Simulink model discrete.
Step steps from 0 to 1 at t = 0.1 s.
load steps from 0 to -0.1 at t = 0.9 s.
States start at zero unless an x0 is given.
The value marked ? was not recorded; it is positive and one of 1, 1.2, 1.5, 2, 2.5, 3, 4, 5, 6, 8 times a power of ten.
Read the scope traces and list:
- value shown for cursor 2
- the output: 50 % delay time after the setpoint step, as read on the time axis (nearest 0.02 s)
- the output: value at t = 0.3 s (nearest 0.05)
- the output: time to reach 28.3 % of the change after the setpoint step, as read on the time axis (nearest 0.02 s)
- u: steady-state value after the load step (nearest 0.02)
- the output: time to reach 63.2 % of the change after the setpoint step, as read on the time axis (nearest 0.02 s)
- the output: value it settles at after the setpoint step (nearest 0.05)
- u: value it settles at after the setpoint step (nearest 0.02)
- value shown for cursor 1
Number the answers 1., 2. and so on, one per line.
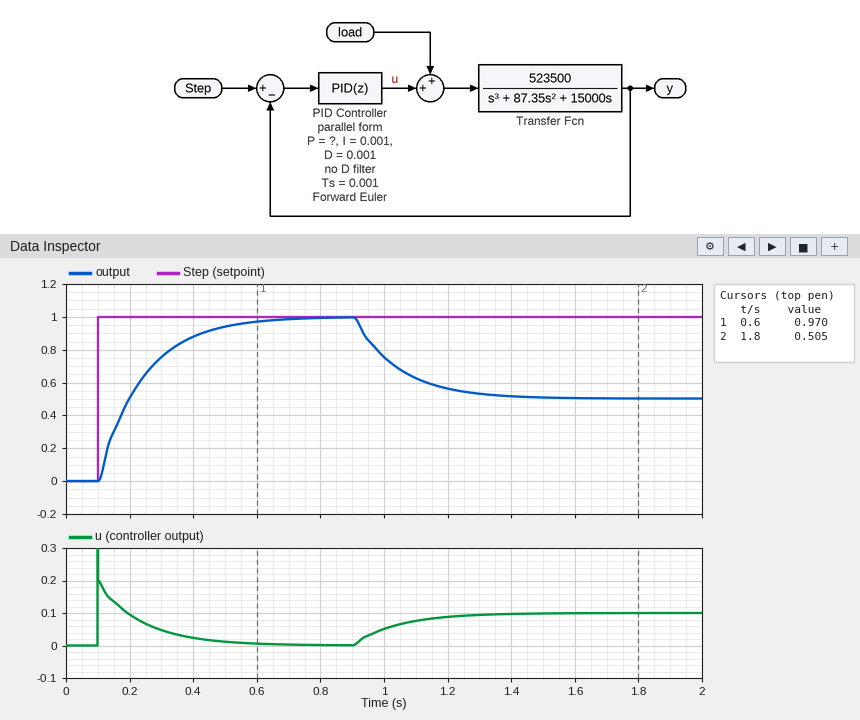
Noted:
1. 0.505
2. 0.20 s
3. 0.75
4. 0.14 s
5. 0.10
6. 0.24 s
7. 1.00
8. 0.00
9. 0.970
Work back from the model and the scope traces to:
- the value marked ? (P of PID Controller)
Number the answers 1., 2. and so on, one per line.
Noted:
1. 0.2
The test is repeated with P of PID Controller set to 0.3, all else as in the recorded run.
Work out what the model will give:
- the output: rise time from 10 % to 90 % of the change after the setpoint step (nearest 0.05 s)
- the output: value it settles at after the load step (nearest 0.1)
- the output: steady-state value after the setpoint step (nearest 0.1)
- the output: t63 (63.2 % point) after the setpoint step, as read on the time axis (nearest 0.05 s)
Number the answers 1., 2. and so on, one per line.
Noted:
1. 0.20 s
2. 0.7
3. 1.0
4. 0.20 s
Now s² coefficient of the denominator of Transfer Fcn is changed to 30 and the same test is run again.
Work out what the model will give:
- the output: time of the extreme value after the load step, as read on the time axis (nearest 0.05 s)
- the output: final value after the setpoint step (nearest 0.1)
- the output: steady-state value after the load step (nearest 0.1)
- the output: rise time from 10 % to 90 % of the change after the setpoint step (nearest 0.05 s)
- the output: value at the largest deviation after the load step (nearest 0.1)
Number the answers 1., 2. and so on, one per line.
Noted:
1. 1.95 s
2. 1.0
3. 0.5
4. 0.30 s
5. 0.5
